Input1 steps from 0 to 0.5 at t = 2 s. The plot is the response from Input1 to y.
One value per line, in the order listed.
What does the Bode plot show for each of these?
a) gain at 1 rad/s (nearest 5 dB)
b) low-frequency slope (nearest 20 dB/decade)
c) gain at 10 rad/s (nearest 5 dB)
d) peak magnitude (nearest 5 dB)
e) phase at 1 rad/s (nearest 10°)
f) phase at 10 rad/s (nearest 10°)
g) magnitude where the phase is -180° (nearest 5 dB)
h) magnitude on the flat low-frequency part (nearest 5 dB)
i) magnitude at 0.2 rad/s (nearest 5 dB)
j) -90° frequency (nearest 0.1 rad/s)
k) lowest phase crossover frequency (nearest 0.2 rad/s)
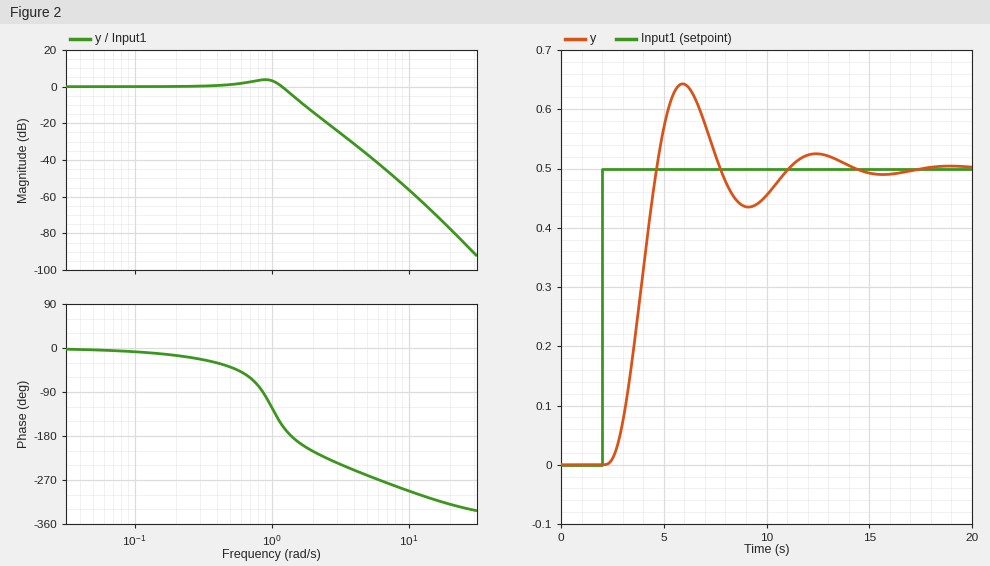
5 dB
0 dB/decade
-55 dB
5 dB
-120°
-290°
-5 dB
0 dB
0 dB
0.9 rad/s
1.4 rad/s
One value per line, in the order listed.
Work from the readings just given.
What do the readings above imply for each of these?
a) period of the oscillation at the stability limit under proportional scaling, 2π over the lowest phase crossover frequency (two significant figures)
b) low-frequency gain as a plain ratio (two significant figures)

4.5 s
1.0
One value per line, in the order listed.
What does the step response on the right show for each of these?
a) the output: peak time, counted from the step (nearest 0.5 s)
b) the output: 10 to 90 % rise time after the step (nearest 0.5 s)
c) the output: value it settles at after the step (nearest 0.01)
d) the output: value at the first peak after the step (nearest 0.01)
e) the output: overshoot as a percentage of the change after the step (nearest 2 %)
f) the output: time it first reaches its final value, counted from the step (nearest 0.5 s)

4.0 s
1.5 s
0.50
0.64
28 %
2.5 s
